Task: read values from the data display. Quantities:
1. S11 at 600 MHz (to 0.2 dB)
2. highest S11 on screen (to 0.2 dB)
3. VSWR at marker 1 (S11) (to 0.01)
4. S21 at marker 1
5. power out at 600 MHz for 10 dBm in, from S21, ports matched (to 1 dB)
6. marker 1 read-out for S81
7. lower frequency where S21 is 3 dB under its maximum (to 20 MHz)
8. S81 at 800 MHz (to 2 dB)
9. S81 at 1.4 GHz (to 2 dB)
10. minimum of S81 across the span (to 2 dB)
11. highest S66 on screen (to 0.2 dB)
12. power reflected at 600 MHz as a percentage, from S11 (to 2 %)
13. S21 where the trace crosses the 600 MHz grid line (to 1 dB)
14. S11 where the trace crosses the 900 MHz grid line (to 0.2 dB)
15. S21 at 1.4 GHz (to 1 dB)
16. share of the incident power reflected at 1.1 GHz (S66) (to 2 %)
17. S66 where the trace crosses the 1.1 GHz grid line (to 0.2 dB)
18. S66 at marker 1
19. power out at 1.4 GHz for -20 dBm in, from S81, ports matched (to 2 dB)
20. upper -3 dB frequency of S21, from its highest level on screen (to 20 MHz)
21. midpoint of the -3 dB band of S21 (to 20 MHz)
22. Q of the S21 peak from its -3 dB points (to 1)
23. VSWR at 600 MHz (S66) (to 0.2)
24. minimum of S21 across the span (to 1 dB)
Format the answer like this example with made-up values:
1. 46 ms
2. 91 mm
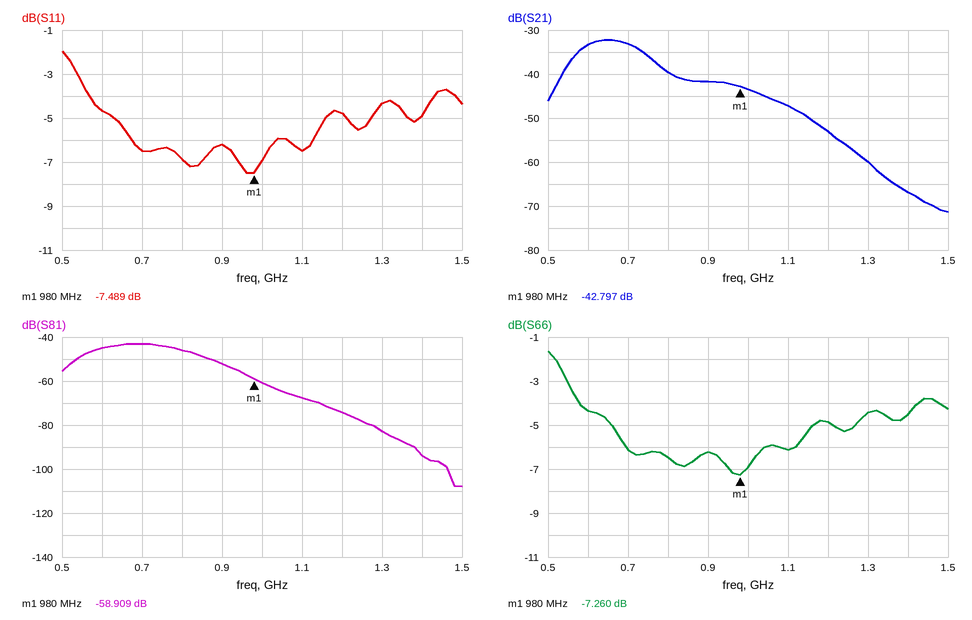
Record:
1. -4.6 dB
2. -2.0 dB
3. 2.46
4. -42.797 dB
5. -23 dBm
6. -58.909 dB
7. 580 MHz
8. -46 dB
9. -94 dB
10. -108 dB
11. -1.6 dB
12. 34 %
13. -33 dB
14. -6.2 dB
15. -67 dB
16. 24 %
17. -6.2 dB
18. -7.260 dB
19. -114 dBm
20. 740 MHz
21. 660 MHz
22. 4
23. 4.0
24. -71 dB
